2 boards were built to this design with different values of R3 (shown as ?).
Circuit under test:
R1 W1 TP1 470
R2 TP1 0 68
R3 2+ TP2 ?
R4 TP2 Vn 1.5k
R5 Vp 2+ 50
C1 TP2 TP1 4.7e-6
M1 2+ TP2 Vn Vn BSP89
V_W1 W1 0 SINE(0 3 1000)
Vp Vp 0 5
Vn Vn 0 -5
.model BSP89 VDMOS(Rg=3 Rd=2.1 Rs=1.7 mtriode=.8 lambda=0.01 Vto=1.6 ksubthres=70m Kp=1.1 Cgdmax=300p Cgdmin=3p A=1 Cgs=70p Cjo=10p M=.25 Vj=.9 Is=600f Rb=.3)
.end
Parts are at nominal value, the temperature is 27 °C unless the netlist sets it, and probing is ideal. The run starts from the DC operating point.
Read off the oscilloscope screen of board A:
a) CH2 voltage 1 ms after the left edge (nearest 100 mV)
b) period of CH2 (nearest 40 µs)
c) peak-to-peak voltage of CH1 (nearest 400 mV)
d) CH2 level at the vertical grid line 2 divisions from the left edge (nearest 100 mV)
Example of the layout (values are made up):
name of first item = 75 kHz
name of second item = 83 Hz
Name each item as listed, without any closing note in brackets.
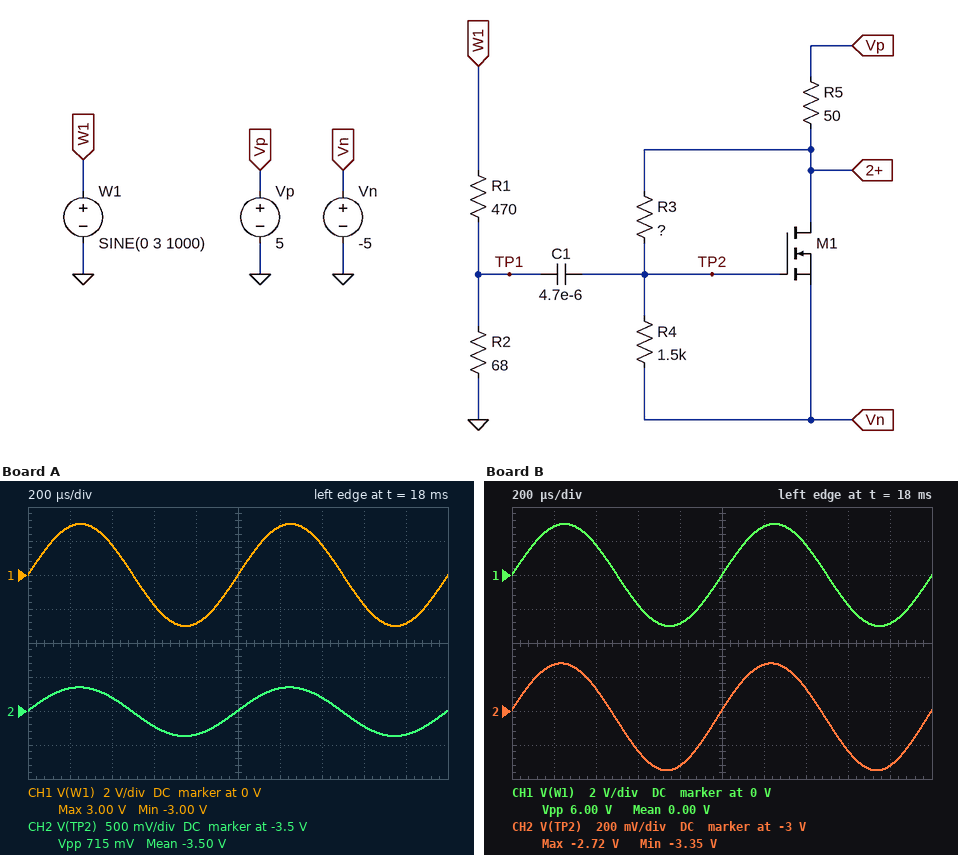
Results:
CH2 voltage 1 ms after the left edge = -3.5 V
period of CH2 = 1.00 ms
peak-to-peak voltage of CH1 = 6.0 V
CH2 level at the vertical grid line 2 divisions from the left edge = -3.3 V
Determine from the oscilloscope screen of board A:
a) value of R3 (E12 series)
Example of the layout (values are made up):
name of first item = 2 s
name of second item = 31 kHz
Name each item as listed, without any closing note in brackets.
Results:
value of R3 = 8.2 kΩ
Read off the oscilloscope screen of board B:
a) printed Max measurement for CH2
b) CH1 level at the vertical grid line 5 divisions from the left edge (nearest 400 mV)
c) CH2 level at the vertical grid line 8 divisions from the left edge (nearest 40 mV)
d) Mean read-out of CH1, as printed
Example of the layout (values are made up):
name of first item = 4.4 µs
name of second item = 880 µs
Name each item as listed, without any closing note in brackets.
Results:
printed Max measurement for CH2 = -2.72 V
CH1 level at the vertical grid line 5 divisions from the left edge = 0 V
CH2 level at the vertical grid line 8 divisions from the left edge = -3.24 V
Mean read-out of CH1, as printed = 0.00 V
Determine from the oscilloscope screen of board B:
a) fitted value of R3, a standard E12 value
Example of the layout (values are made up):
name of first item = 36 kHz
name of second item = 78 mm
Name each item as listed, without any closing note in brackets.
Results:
fitted value of R3, a standard E12 value = 3.9 kΩ
